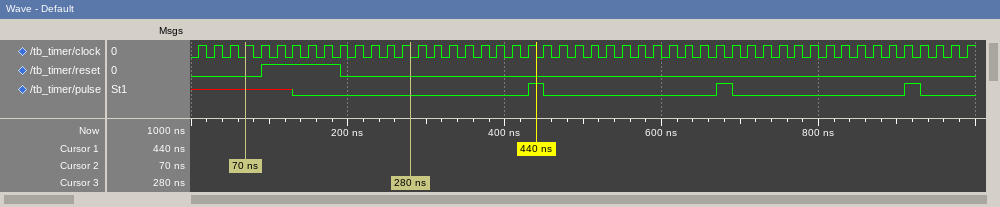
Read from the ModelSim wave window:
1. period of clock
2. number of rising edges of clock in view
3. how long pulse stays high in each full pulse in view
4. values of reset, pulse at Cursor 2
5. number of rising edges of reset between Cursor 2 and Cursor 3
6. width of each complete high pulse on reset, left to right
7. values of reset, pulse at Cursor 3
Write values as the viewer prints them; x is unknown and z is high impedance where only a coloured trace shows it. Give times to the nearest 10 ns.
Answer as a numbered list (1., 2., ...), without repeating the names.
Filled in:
1. 20 ns
2. 50
3. 20 ns, 20 ns, 20 ns
4. reset=0, pulse=x
5. 1
6. 100 ns
7. reset=0, pulse=0
